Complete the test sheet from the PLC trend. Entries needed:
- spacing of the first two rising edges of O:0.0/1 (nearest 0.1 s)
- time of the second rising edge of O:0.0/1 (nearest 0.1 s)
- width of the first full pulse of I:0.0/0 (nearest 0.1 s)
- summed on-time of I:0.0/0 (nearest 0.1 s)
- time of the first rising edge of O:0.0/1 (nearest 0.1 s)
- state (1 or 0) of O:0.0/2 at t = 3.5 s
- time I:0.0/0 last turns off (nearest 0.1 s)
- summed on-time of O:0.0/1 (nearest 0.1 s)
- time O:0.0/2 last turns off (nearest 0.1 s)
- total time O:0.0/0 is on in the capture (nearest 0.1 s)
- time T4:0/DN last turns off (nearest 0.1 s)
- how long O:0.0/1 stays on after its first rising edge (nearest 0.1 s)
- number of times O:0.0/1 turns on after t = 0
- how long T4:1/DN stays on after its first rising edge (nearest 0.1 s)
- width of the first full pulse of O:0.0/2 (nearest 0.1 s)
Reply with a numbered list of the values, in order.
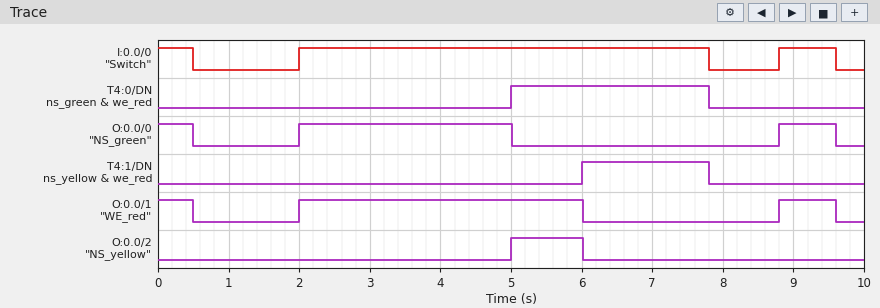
1. 6.8 s
2. 8.8 s
3. 5.8 s
4. 7.1 s
5. 2.0 s
6. 0
7. 9.6 s
8. 5.3 s
9. 6.0 s
10. 4.3 s
11. 7.8 s
12. 4.0 s
13. 2
14. 1.8 s
15. 1.0 s
